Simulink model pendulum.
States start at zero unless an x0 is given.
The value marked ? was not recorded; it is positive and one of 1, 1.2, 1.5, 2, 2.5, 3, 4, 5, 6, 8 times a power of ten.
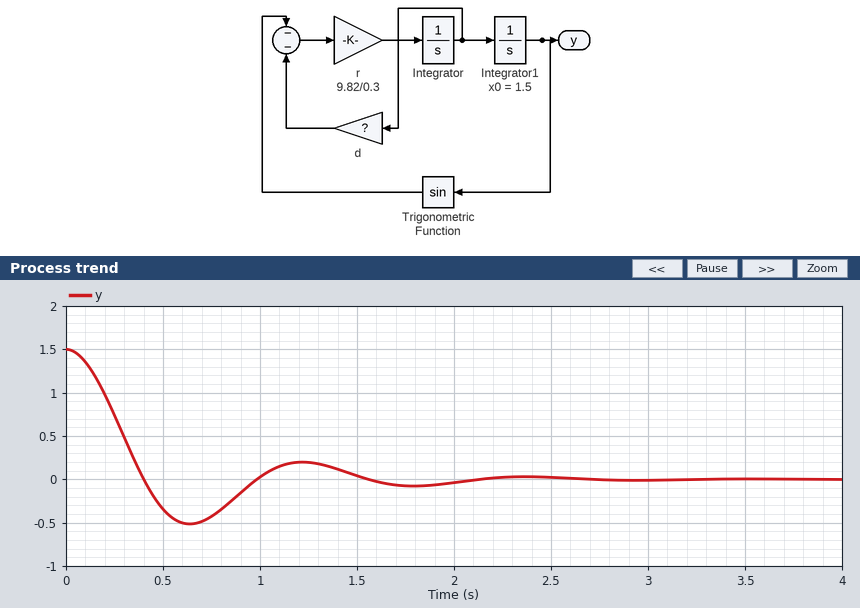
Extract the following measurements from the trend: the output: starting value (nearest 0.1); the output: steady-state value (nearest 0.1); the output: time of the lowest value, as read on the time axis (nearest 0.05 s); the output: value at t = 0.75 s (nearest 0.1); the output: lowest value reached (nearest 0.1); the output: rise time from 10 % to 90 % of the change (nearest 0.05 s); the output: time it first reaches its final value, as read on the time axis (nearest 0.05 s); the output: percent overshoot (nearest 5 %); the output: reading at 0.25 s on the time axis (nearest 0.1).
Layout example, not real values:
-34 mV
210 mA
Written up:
1.5
0.0
0.65 s
-0.4
-0.5
0.25 s
0.40 s
35 %
0.7
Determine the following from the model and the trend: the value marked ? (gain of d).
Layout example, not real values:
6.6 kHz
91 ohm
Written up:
0.1
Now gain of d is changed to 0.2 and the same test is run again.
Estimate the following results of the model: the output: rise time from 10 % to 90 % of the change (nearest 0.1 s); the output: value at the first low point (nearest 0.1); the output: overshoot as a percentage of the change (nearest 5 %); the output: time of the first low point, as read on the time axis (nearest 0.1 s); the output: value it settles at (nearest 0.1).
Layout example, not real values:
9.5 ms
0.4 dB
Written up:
0.4 s
-0.1
10 %
0.8 s
0.0
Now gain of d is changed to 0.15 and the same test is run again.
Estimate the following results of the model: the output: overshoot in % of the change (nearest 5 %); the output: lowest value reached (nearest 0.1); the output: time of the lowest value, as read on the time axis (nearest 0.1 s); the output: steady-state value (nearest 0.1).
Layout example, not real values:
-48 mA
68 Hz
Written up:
20 %
-0.3
0.7 s
0.0
